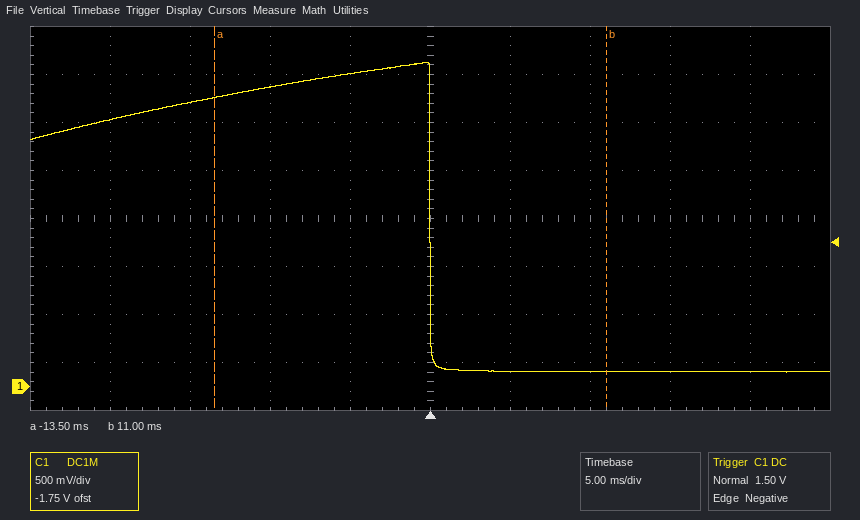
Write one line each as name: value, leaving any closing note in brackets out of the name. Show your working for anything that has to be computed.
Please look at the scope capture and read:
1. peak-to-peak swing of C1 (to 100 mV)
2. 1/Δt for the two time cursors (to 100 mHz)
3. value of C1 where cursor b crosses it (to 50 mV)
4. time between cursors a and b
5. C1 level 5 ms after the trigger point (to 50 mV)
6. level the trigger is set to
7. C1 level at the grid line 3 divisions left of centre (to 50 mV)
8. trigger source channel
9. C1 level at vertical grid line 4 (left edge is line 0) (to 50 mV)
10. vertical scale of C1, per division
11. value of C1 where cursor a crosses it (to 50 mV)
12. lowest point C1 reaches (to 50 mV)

peak-to-peak swing of C1: 3.20 V
1/Δt for the two time cursors: 1 / 24.5 ms ≈ 40.8 Hz
value of C1 where cursor b crosses it: 150 mV
time between cursors a and b: 11 ms − (-13.5 ms) = 24.5 ms
C1 level 5 ms after the trigger point: 150 mV
level the trigger is set to: 1.50 V
C1 level at the grid line 3 divisions left of centre: 2.95 V
trigger source channel: C1
C1 level at vertical grid line 4 (left edge is line 0): 3.25 V
vertical scale of C1, per division: 500 mV
value of C1 where cursor a crosses it: 3.00 V
lowest point C1 reaches: 150 mV
